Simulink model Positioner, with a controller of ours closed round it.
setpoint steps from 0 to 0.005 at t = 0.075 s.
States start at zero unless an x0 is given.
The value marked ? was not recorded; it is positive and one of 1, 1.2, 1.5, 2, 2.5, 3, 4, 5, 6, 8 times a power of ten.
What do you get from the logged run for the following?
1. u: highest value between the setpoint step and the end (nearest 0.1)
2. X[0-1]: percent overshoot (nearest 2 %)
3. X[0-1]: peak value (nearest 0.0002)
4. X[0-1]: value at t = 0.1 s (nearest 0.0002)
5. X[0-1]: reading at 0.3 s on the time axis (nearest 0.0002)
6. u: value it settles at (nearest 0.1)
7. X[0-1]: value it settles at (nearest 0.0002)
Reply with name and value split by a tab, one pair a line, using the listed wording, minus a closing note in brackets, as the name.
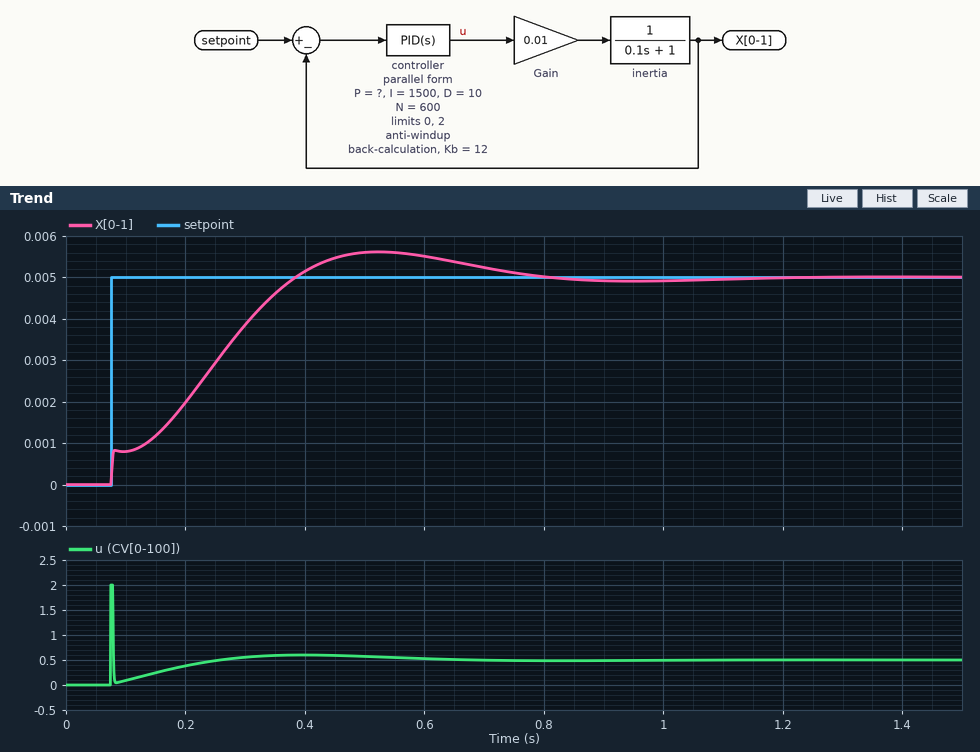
u: highest value between the setpoint step and the end	2.0
X[0-1]: percent overshoot	12 %
X[0-1]: peak value	0.0056
X[0-1]: value at t = 0.1 s	0.0008
X[0-1]: reading at 0.3 s on the time axis	0.0038
u: value it settles at	0.5
X[0-1]: value it settles at	0.0050
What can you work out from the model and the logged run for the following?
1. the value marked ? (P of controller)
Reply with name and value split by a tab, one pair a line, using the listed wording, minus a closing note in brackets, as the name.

the value marked ?	80
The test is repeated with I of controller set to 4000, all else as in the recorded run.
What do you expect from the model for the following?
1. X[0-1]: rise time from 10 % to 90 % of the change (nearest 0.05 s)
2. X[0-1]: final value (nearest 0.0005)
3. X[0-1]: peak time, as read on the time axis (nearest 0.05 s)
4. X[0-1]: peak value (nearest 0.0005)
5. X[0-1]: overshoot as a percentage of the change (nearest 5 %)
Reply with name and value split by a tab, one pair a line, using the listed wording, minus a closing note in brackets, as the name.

X[0-1]: rise time from 10 % to 90 % of the change	0.15 s
X[0-1]: final value	0.0050
X[0-1]: peak time, as read on the time axis	0.30 s
X[0-1]: peak value	0.0065
X[0-1]: overshoot as a percentage of the change	30 %
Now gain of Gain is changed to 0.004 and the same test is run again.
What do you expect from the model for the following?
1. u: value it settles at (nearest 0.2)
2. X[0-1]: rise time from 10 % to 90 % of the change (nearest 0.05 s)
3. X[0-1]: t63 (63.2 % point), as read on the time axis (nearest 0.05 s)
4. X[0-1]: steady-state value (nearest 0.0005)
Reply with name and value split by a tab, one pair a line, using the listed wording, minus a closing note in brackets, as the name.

u: value it settles at	1.2
X[0-1]: rise time from 10 % to 90 % of the change	0.35 s
X[0-1]: t63 (63.2 % point), as read on the time axis	0.35 s
X[0-1]: steady-state value	0.0050
